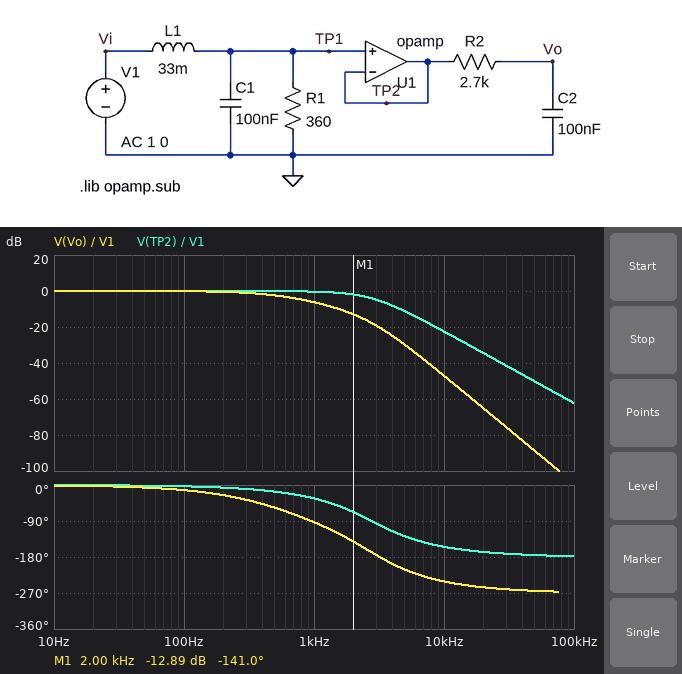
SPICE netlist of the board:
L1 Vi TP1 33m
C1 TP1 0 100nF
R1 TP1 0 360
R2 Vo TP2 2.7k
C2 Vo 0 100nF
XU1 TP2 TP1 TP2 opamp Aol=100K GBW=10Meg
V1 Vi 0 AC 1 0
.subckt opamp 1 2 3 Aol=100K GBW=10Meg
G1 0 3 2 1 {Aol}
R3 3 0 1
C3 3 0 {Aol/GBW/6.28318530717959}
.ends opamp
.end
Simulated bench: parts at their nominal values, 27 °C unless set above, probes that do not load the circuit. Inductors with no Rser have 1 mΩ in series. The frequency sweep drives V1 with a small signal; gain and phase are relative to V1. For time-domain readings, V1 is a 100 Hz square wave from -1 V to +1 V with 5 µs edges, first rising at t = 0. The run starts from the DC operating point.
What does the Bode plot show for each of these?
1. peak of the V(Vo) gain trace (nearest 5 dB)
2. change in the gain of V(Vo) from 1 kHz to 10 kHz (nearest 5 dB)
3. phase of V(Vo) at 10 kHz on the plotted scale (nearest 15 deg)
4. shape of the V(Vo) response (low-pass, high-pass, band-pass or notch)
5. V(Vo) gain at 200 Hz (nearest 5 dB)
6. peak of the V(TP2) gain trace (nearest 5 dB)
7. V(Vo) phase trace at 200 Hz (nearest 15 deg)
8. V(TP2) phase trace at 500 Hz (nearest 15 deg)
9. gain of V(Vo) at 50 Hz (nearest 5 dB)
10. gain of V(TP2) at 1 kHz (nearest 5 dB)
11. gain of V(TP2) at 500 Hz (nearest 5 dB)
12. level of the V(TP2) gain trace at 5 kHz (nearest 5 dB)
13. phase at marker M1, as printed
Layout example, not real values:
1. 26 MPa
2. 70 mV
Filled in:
1. 0 dB
2. -40 dB
3. -240 deg
4. low-pass
5. 0 dB
6. 0 dB
7. -30 deg
8. -15 deg
9. 0 dB
10. 0 dB
11. 0 dB
12. -10 dB
13. -141.0 deg
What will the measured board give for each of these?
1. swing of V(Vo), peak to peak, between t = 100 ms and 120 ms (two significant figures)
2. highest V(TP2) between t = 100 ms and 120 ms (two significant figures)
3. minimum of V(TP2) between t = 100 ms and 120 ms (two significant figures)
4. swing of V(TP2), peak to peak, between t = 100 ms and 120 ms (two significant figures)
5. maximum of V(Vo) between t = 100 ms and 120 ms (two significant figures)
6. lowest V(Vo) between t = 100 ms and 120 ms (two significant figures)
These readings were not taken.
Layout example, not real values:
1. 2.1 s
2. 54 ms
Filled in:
1. 2.0 V
2. 1.0 V
3. -1.0 V
4. 2.1 V
5. 1.0 V
6. -1.0 V
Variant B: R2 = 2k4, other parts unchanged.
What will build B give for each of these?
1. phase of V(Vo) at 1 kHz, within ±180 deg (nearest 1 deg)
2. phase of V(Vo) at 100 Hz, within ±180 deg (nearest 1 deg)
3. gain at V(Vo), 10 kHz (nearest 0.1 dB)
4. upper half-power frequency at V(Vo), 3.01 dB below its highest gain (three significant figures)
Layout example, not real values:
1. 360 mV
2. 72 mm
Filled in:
1. -90 deg
2. -12 deg
3. -46.1 dB
4. 642 Hz
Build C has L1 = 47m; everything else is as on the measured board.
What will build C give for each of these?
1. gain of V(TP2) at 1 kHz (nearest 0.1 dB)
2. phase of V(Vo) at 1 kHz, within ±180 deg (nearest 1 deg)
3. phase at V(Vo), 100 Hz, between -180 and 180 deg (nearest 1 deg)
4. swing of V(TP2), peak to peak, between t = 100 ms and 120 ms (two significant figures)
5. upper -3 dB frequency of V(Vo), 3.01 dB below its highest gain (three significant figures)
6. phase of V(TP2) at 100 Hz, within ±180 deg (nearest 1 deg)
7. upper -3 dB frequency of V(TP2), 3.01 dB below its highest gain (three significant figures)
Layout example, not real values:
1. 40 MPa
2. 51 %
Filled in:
1. -1.3 dB
2. -105 deg
3. -14 deg
4. 2.0 V
5. 538 Hz
6. -5 deg
7. 1.60 kHz
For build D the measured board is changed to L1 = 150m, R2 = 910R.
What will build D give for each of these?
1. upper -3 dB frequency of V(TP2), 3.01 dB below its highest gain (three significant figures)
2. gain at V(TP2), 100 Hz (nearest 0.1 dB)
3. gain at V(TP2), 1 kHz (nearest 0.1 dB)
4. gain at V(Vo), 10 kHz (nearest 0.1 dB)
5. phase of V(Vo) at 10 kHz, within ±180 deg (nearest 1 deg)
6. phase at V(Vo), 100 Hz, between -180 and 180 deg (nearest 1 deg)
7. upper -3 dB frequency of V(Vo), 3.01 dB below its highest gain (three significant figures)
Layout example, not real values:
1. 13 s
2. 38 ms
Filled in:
1. 418 Hz
2. -0.2 dB
3. -8.5 dB
4. -51.4 dB
5. 124 deg
6. -18 deg
7. 397 Hz
